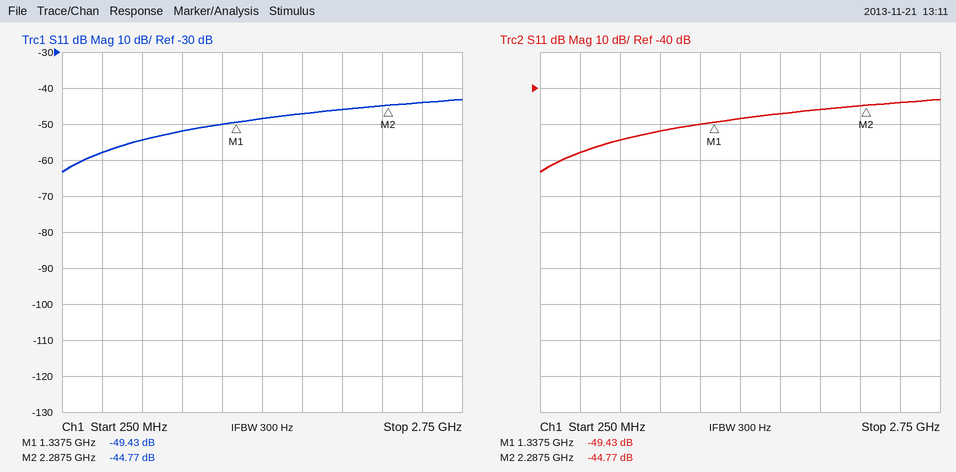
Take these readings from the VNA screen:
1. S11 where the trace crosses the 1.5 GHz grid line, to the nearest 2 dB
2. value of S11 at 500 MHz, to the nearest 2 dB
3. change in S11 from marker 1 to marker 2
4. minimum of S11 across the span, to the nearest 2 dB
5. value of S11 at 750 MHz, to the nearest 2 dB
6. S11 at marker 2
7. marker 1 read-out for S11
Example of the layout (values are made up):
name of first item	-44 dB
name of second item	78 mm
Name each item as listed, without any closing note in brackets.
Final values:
S11 where the trace crosses the 1.5 GHz grid line, to the nearest 2 dB	-48 dB
value of S11 at 500 MHz, to the nearest 2 dB	-58 dB
change in S11 from marker 1 to marker 2	4.66 dB
minimum of S11 across the span, to the nearest 2 dB	-64 dB
value of S11 at 750 MHz, to the nearest 2 dB	-54 dB
S11 at marker 2	-44.77 dB
marker 1 read-out for S11	-49.43 dB
